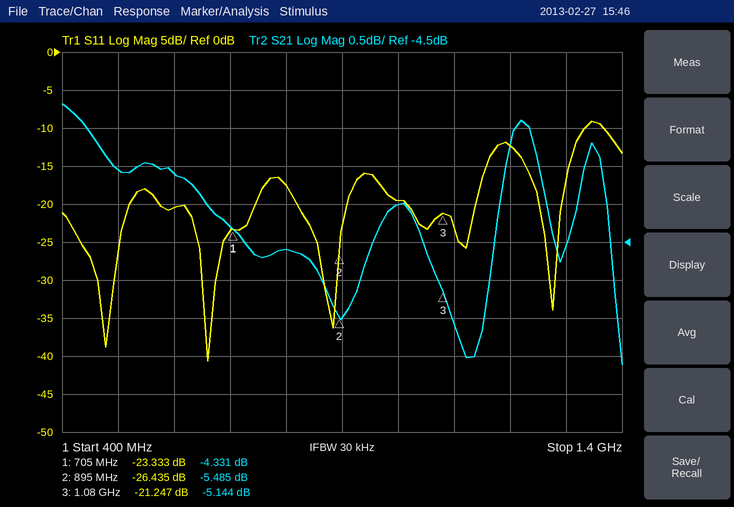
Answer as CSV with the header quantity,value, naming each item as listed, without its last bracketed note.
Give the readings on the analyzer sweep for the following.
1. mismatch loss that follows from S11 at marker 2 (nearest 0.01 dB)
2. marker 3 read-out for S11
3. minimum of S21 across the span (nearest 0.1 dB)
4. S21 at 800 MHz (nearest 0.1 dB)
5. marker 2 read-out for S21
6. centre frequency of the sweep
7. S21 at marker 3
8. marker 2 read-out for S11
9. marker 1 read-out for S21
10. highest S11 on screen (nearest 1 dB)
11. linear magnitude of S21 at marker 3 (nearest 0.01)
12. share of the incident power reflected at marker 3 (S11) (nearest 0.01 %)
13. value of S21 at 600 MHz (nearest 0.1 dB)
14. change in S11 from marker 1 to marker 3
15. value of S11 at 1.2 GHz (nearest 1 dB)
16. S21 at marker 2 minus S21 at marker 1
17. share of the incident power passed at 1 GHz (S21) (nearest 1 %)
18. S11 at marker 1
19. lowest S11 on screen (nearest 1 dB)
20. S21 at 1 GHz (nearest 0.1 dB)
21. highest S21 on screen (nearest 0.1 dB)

quantity,value
mismatch loss that follows from S11 at marker 2,0.01 dB
marker 3 read-out for S11,-21.247 dB
minimum of S21 across the span,-6.1 dB
S21 at 800 MHz,-4.6 dB
marker 2 read-out for S21,-5.485 dB
centre frequency of the sweep,900 MHz
S21 at marker 3,-5.144 dB
marker 2 read-out for S11,-26.435 dB
marker 1 read-out for S21,-4.331 dB
highest S11 on screen,-9 dB
linear magnitude of S21 at marker 3,0.55
share of the incident power reflected at marker 3 (S11),0.75 %
value of S21 at 600 MHz,-3.6 dB
change in S11 from marker 1 to marker 3,2.086 dB
value of S11 at 1.2 GHz,-12 dB
S21 at marker 2 minus S21 at marker 1,-1.154 dB
share of the incident power passed at 1 GHz (S21),40 %
S11 at marker 1,-23.333 dB
lowest S11 on screen,-41 dB
S21 at 1 GHz,-4.0 dB
highest S21 on screen,-2.7 dB
